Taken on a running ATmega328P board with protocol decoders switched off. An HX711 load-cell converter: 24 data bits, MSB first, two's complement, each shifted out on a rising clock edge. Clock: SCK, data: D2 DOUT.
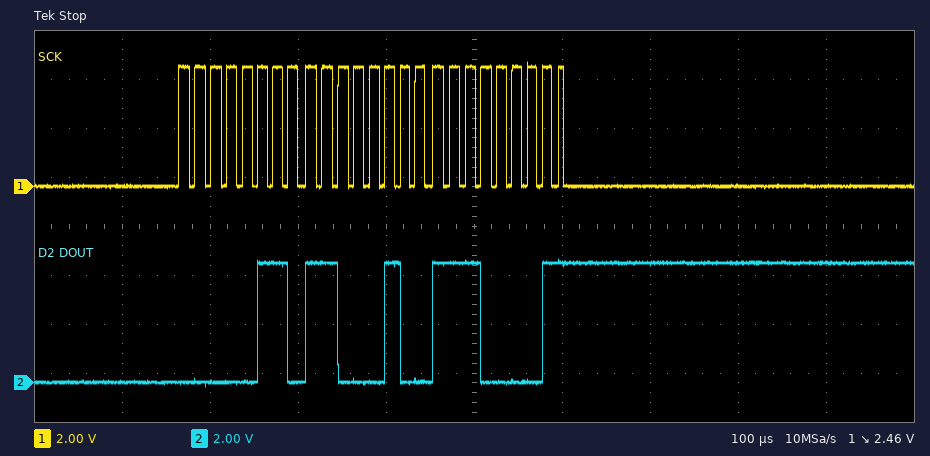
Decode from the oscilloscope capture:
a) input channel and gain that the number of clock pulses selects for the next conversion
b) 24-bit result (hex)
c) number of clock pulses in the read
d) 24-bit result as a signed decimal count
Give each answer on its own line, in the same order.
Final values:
channel A, gain 128
0x06C4E1
25
443617
